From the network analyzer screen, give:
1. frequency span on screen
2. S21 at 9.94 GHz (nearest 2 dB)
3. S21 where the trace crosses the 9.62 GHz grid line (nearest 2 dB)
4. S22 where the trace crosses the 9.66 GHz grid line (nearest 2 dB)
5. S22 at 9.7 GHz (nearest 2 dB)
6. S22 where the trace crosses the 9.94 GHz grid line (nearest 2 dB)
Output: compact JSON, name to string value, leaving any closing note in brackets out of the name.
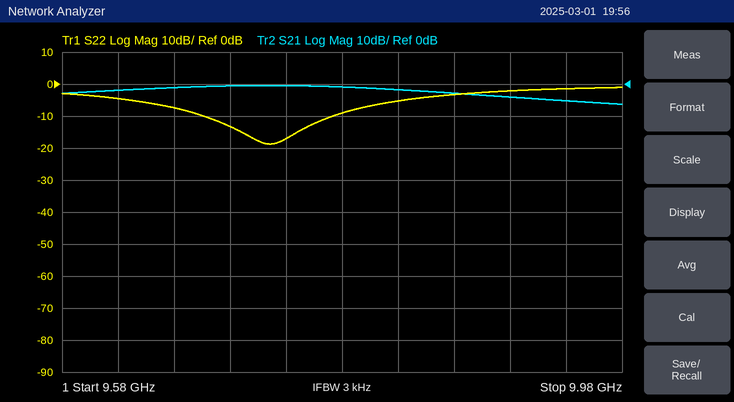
{"frequency span on screen": "400 MHz", "S21 at 9.94 GHz": "-6 dB", "S21 where the trace crosses the 9.62 GHz grid line": "-2 dB", "S22 where the trace crosses the 9.66 GHz grid line": "-8 dB", "S22 at 9.7 GHz": "-14 dB", "S22 where the trace crosses the 9.94 GHz grid line": "-2 dB"}
